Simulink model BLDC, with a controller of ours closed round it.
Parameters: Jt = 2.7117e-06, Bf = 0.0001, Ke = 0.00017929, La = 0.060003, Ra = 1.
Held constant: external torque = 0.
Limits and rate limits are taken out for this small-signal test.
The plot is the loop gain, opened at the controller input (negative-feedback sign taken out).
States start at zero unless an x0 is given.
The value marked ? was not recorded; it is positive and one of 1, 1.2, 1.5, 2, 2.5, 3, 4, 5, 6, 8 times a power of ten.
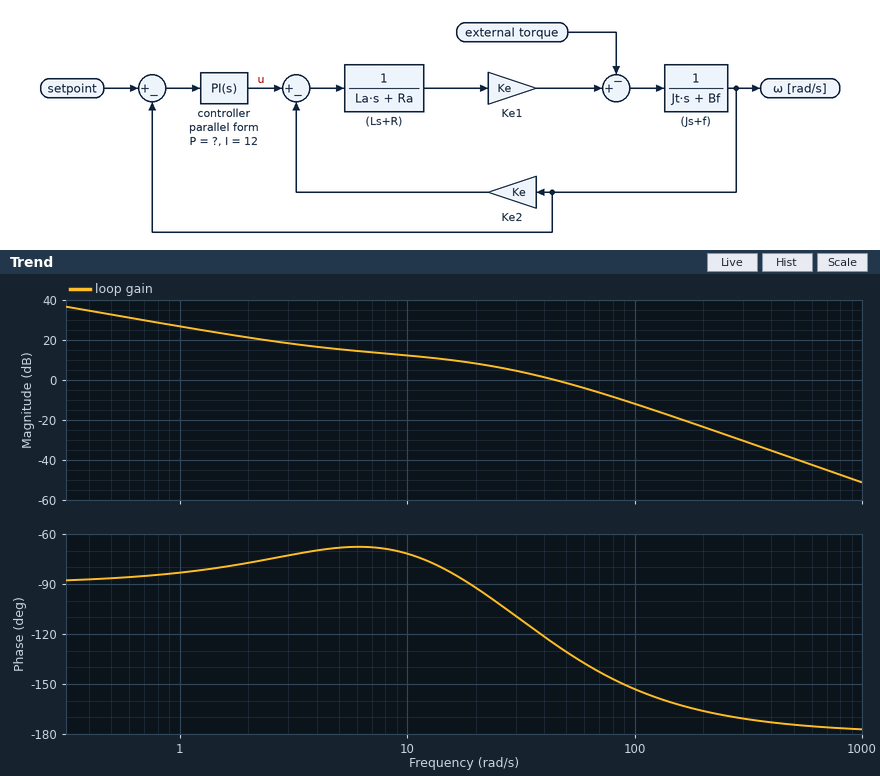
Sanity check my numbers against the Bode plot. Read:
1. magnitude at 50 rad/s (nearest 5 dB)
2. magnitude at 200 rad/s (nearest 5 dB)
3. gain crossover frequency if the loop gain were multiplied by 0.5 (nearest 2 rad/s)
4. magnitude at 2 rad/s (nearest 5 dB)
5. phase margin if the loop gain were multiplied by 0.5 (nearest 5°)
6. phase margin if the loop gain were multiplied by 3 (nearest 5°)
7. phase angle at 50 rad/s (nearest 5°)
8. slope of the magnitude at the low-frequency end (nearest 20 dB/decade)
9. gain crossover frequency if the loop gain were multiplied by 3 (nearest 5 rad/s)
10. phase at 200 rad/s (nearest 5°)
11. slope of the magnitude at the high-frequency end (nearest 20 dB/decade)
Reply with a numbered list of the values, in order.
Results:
1. 0 dB
2. -25 dB
3. 26 rad/s
4. 20 dB
5. 75°
6. 30°
7. -130°
8. -20 dB/decade
9. 85 rad/s
10. -165°
11. -40 dB/decade
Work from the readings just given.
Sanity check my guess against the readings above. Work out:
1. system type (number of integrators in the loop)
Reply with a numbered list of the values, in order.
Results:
1. 1
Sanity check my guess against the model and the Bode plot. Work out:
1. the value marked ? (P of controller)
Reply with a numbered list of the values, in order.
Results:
1. 2.5
